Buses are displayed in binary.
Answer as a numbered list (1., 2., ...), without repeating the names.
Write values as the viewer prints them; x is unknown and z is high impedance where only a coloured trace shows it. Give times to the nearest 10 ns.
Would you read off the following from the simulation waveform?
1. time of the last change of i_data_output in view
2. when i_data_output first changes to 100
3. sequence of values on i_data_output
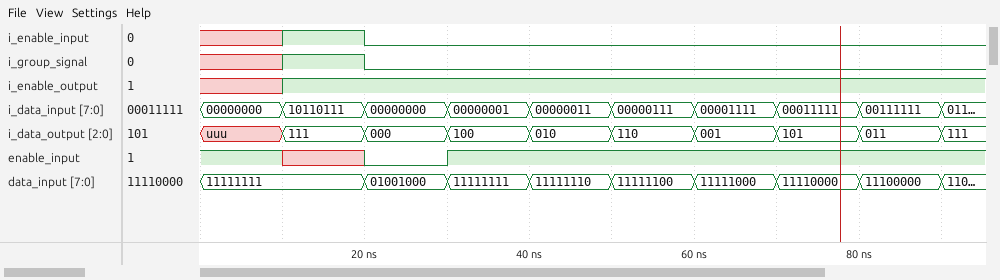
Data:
1. 90 ns
2. 30 ns
3. uuu, 111, 000, 100, 010, 110, 001, 101, 011, 111
